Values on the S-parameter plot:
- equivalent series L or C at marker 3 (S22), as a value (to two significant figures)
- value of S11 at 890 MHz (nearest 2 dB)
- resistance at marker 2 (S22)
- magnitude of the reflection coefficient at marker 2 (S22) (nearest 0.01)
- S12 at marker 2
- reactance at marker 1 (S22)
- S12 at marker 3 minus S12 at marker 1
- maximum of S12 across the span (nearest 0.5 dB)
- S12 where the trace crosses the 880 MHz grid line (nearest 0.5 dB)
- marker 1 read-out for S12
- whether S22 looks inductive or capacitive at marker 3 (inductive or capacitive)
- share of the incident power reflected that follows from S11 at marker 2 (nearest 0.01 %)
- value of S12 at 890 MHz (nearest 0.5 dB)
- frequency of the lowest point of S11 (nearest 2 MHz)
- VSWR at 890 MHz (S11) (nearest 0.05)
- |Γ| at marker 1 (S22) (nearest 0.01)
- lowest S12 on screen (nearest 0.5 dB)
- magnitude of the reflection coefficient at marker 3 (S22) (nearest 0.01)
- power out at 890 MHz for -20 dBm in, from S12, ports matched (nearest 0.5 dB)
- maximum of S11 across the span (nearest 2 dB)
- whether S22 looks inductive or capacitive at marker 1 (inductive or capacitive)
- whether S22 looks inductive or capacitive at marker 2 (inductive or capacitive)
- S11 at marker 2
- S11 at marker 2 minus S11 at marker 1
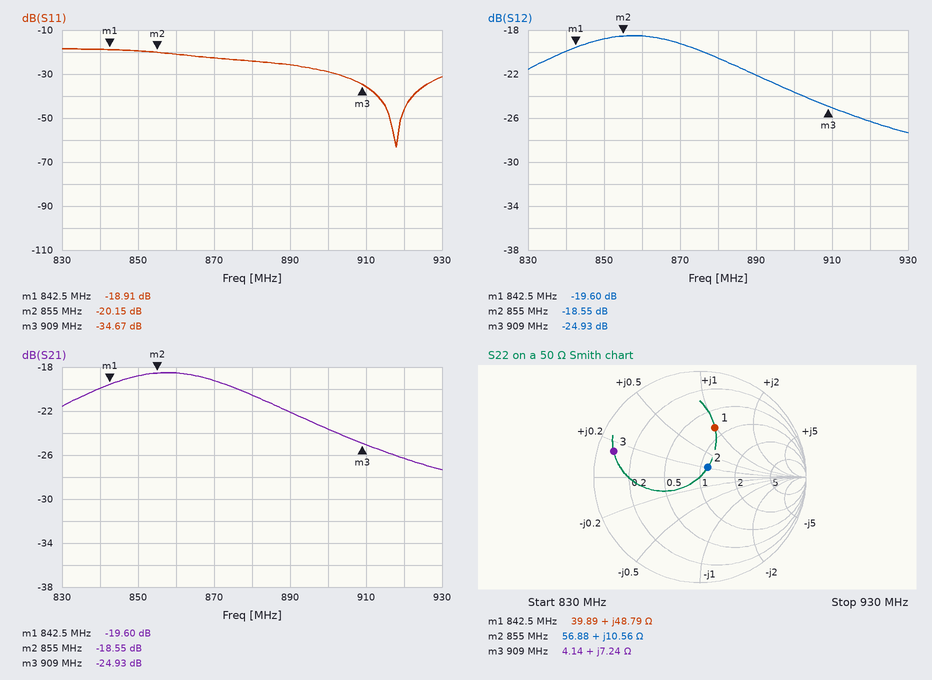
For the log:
1.3 nH
-26 dB
56.88 Ω
0.12
-18.55 dB
+48.79 Ω
-5.33 dB
-18.5 dB
-20.5 dB
-19.60 dB
inductive
0.97 %
-22.0 dB
918 MHz
1.10
0.49
-27.5 dB
0.85
-42.0 dBm
-18 dB
inductive
inductive
-20.15 dB
-1.24 dB
